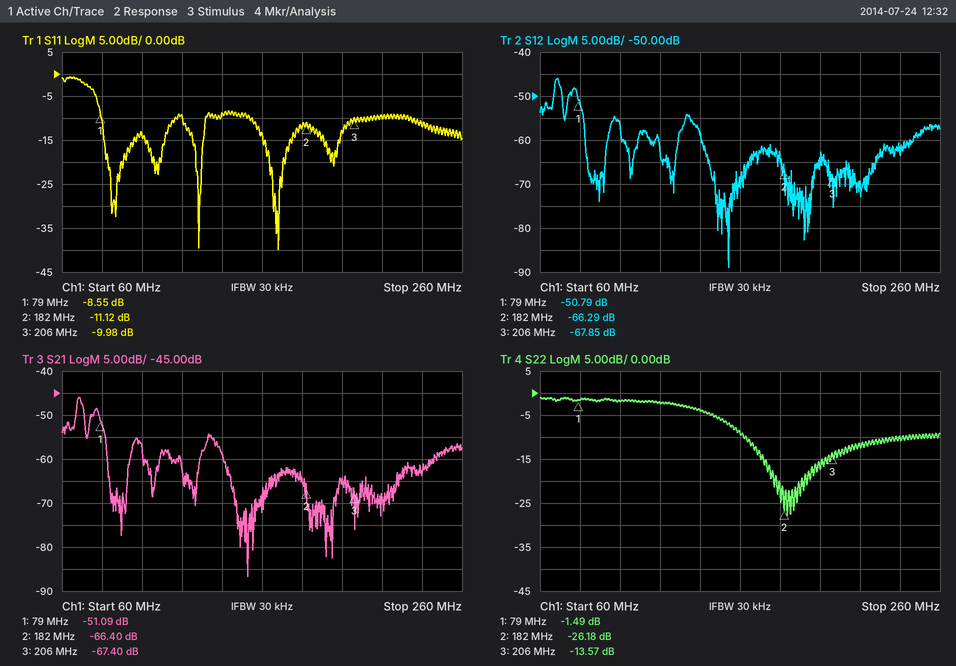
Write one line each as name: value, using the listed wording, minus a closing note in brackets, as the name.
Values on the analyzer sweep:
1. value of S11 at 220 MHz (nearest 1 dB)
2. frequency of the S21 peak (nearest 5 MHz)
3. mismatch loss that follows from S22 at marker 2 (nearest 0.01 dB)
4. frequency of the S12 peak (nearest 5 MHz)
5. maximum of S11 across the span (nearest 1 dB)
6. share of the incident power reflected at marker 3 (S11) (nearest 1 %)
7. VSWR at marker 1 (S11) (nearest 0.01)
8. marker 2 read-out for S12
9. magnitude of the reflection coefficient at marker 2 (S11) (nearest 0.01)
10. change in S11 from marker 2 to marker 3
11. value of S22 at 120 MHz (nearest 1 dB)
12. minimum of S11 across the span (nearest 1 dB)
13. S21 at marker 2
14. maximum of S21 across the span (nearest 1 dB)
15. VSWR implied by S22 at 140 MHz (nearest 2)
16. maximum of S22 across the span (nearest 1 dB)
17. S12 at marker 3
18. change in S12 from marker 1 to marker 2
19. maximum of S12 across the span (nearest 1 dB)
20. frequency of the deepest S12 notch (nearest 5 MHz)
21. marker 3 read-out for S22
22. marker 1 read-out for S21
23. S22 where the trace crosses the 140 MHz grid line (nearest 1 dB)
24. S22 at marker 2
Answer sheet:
value of S11 at 220 MHz: -10 dB
frequency of the S21 peak: 70 MHz
mismatch loss that follows from S22 at marker 2: 0.01 dB
frequency of the S12 peak: 70 MHz
maximum of S11 across the span: -1 dB
share of the incident power reflected at marker 3 (S11): 10 %
VSWR at marker 1 (S11): 2.19
marker 2 read-out for S12: -66.29 dB
magnitude of the reflection coefficient at marker 2 (S11): 0.28
change in S11 from marker 2 to marker 3: 1.14 dB
value of S22 at 120 MHz: -2 dB
minimum of S11 across the span: -40 dB
S21 at marker 2: -66.40 dB
maximum of S21 across the span: -46 dB
VSWR implied by S22 at 140 MHz: 4
maximum of S22 across the span: -1 dB
S12 at marker 3: -67.85 dB
change in S12 from marker 1 to marker 2: -15.50 dB
maximum of S12 across the span: -46 dB
frequency of the deepest S12 notch: 155 MHz
marker 3 read-out for S22: -13.57 dB
marker 1 read-out for S21: -51.09 dB
S22 where the trace crosses the 140 MHz grid line: -4 dB
S22 at marker 2: -26.18 dB
